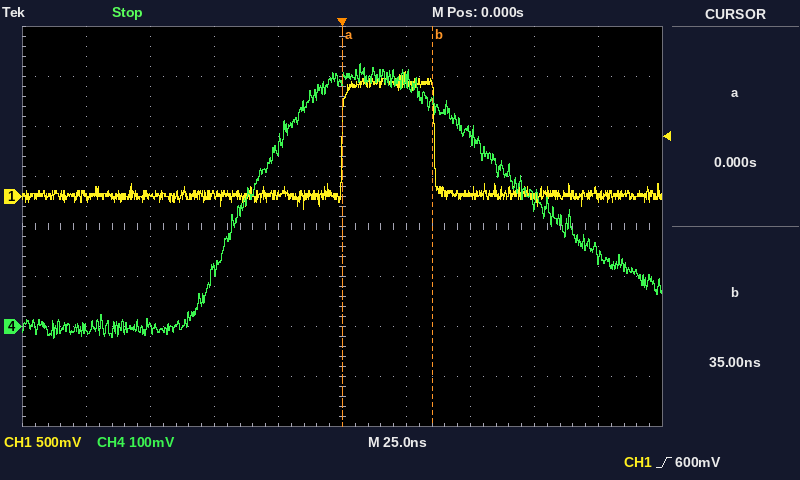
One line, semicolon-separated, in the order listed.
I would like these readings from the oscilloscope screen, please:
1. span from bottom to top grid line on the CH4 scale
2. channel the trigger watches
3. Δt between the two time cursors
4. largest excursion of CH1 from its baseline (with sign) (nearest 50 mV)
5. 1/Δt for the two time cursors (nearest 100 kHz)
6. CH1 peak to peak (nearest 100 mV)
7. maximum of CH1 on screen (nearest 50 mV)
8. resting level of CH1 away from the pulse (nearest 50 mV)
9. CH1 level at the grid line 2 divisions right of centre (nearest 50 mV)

800 mV; CH1; 35.0 ns; +1.25 V; 28.6 MHz; 1.40 V; 1.25 V; 0 mV; 0 mV
